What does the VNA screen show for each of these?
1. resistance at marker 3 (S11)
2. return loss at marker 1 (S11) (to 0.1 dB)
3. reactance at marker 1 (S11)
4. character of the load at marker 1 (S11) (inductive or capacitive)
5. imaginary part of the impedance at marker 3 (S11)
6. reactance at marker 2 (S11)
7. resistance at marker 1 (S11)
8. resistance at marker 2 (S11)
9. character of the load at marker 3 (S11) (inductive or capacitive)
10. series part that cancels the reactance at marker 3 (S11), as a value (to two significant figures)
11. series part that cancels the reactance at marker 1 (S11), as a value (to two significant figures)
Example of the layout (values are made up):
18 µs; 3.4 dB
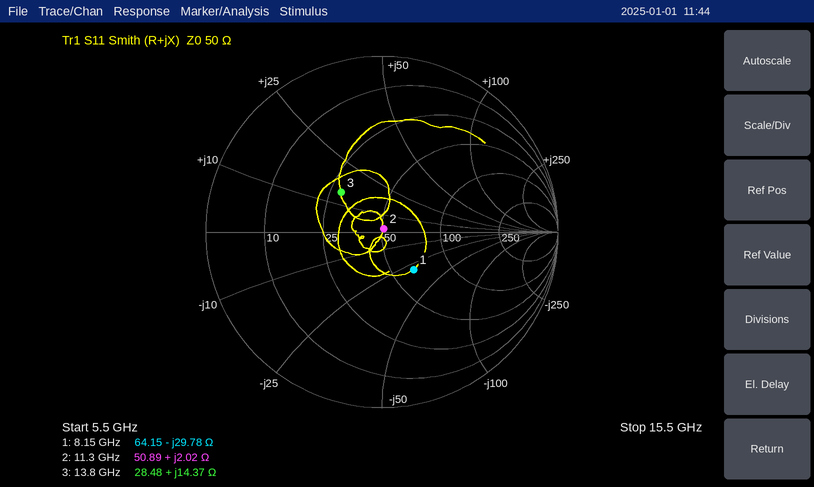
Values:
28.48 Ω; 11.1 dB; -29.78 Ω; capacitive; +14.37 Ω; +2.02 Ω; 64.15 Ω; 50.89 Ω; inductive; 800 fF; 580 pH
